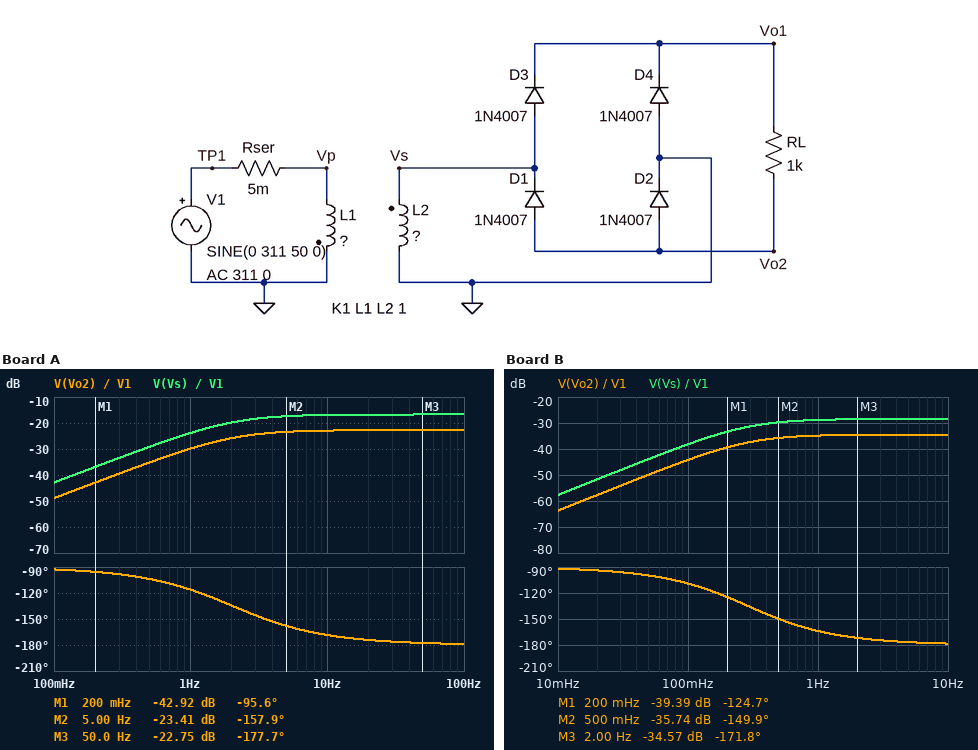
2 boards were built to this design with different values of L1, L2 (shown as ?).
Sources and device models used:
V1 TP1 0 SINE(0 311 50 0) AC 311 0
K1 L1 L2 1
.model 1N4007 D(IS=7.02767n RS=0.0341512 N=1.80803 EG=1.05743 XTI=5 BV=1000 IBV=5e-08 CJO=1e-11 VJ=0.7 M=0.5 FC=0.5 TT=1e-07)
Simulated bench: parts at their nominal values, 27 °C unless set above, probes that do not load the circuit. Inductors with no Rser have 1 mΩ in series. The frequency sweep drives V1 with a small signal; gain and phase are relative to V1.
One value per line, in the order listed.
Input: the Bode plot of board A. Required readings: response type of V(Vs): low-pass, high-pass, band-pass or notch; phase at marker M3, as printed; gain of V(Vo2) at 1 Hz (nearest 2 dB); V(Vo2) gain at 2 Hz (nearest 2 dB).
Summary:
high-pass
-177.7 deg
-30 dB
-26 dB
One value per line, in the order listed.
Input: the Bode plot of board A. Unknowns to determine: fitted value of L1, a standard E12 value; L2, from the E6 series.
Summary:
470 µH
10 µH
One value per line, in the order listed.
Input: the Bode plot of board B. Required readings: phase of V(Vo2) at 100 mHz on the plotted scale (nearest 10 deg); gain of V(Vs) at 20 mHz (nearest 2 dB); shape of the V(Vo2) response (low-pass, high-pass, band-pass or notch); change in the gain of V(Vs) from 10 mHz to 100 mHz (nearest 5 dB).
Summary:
-110 deg
-52 dB
high-pass
20 dB
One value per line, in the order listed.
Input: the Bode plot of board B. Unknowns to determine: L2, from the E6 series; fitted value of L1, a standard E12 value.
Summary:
4.7 µH
3.3 mH
